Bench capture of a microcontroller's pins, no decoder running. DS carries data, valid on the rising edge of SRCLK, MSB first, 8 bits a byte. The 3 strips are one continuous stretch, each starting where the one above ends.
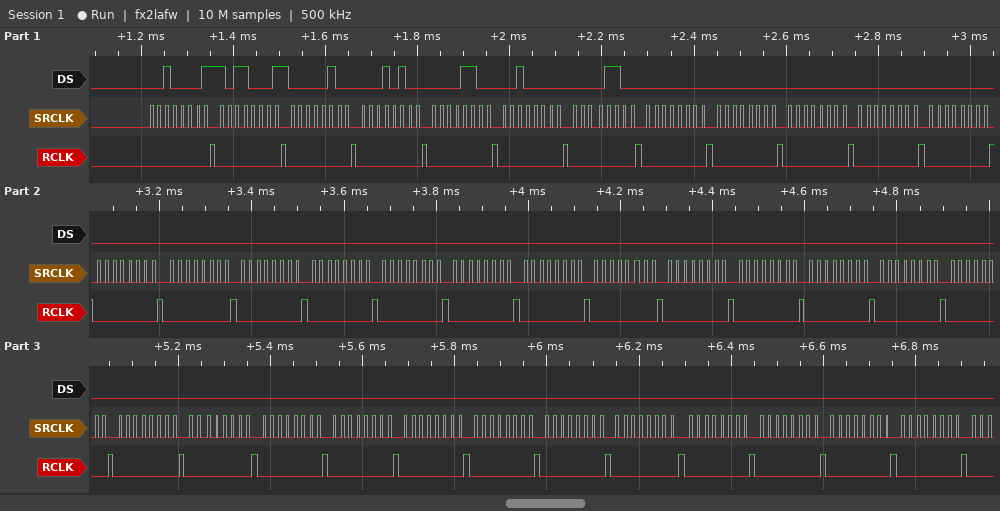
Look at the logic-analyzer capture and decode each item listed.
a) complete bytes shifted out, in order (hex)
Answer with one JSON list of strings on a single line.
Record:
["21 B1 04 14 0C 20 0C 00 00 00 00 00 00 00 00 00 00 00 00 00 00 00 00 00 00 00 00 00 00 00 00 00 00 00 00 00 00"]
